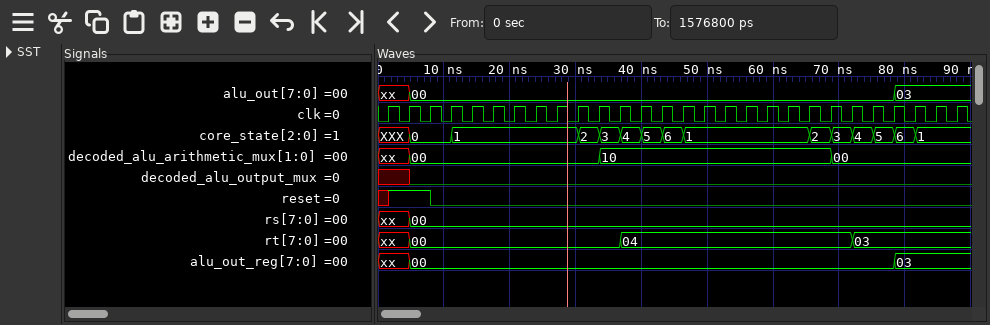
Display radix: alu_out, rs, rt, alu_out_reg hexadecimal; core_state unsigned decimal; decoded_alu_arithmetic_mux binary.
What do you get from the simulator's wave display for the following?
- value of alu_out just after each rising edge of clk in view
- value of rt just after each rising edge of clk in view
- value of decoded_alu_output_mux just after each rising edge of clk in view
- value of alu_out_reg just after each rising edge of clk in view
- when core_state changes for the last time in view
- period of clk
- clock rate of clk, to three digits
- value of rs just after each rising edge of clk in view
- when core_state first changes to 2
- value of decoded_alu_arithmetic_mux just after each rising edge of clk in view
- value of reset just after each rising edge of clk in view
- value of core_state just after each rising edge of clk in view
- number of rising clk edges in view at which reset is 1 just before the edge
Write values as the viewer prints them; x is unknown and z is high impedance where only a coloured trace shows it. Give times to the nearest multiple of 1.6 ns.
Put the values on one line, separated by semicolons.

xx, 00, 00, 00, 00, 00, 00, 00, 00, 00, 00, 00, 00, 00, 00, 00, 00, 00, 00, 00, 00, 00, 00, 00, 03, 03, 03, 03; xx, 00, 00, 00, 00, 00, 00, 00, 00, 00, 00, 04, 04, 04, 04, 04, 04, 04, 04, 04, 04, 04, 03, 03, 03, 03, 03, 03; x 0 0 0 0 0 0 0 0 0 0 0 0 0 0 0 0 0 0 0 0 0 0 0 0 0 0 0; xx, 00, 00, 00, 00, 00, 00, 00, 00, 00, 00, 00, 00, 00, 00, 00, 00, 00, 00, 00, 00, 00, 00, 00, 03, 03, 03, 03; 81.6 ns; 3.2 ns; 312 MHz; xx, 00, 00, 00, 00, 00, 00, 00, 00, 00, 00, 00, 00, 00, 00, 00, 00, 00, 00, 00, 00, 00, 00, 00, 00, 00, 00, 00; 30.4 ns; xx, 00, 00, 00, 00, 00, 00, 00, 00, 00, 10, 10, 10, 10, 10, 10, 10, 10, 10, 10, 10, 00, 00, 00, 00, 00, 00, 00; 1 1 0 0 0 0 0 0 0 0 0 0 0 0 0 0 0 0 0 0 0 0 0 0 0 0 0 0; XXX, 0, 0, 1, 1, 1, 1, 1, 1, 2, 3, 4, 5, 6, 1, 1, 1, 1, 1, 1, 2, 3, 4, 5, 6, 1, 1, 1; 2
